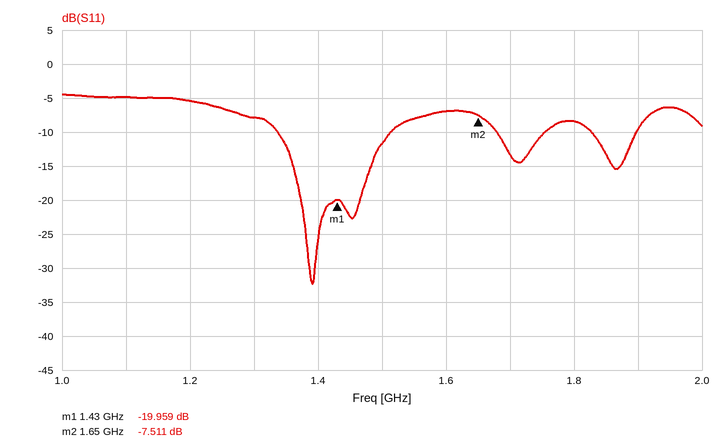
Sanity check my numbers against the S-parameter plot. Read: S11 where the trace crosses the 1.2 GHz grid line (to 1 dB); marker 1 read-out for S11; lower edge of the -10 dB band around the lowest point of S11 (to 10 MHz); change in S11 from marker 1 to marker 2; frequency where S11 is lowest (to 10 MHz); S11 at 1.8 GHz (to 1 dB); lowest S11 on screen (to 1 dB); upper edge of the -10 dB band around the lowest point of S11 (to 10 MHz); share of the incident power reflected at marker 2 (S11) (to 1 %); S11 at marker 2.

-5 dB
-19.959 dB
1.34 GHz
12.448 dB
1.39 GHz
-8 dB
-32 dB
1.51 GHz
18 %
-7.511 dB
